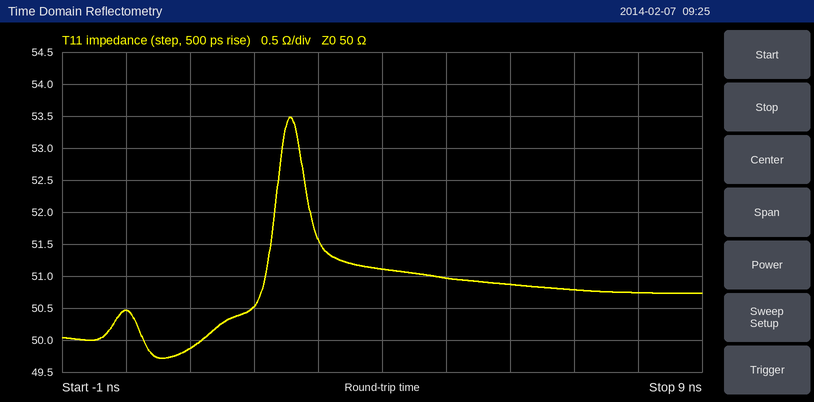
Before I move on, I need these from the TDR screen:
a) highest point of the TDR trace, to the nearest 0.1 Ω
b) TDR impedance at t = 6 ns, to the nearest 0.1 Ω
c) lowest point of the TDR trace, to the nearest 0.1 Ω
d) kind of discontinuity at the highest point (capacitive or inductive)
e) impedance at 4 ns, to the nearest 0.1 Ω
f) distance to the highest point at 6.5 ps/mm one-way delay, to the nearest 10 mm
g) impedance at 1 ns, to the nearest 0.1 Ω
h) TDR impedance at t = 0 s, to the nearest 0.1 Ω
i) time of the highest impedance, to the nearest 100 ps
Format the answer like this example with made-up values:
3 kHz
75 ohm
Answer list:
53.5 Ω
50.9 Ω
49.7 Ω
inductive
51.1 Ω
200 mm
49.9 Ω
50.5 Ω
2.6 ns
